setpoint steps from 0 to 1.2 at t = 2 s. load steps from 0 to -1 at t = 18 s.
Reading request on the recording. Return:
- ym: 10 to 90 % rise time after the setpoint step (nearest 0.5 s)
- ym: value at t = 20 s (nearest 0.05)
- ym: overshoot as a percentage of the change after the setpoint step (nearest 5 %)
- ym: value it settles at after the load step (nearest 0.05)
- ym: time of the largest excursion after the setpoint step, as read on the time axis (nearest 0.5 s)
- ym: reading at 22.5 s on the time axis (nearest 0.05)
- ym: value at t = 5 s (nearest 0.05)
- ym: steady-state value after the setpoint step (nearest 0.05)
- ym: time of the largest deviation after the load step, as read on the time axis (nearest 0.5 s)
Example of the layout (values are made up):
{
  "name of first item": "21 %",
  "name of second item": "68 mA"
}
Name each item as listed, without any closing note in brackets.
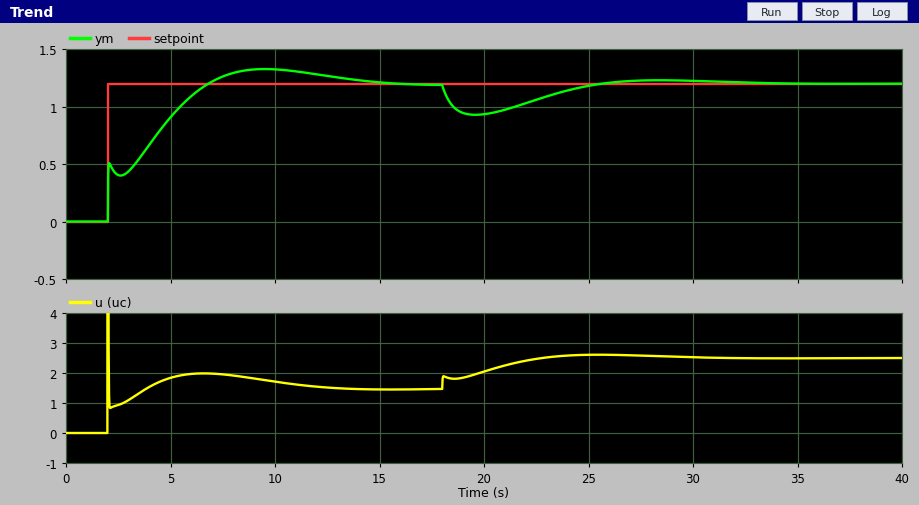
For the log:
{
  "ym: 10 to 90 % rise time after the setpoint step": "4.0 s",
  "ym: value at t = 20 s": "0.95",
  "ym: overshoot as a percentage of the change after the setpoint step": "10 %",
  "ym: value it settles at after the load step": "1.20",
  "ym: time of the largest excursion after the setpoint step, as read on the time axis": "9.5 s",
  "ym: reading at 22.5 s on the time axis": "1.05",
  "ym: value at t = 5 s": "0.90",
  "ym: steady-state value after the setpoint step": "1.20",
  "ym: time of the largest deviation after the load step, as read on the time axis": "19.5 s"
}
